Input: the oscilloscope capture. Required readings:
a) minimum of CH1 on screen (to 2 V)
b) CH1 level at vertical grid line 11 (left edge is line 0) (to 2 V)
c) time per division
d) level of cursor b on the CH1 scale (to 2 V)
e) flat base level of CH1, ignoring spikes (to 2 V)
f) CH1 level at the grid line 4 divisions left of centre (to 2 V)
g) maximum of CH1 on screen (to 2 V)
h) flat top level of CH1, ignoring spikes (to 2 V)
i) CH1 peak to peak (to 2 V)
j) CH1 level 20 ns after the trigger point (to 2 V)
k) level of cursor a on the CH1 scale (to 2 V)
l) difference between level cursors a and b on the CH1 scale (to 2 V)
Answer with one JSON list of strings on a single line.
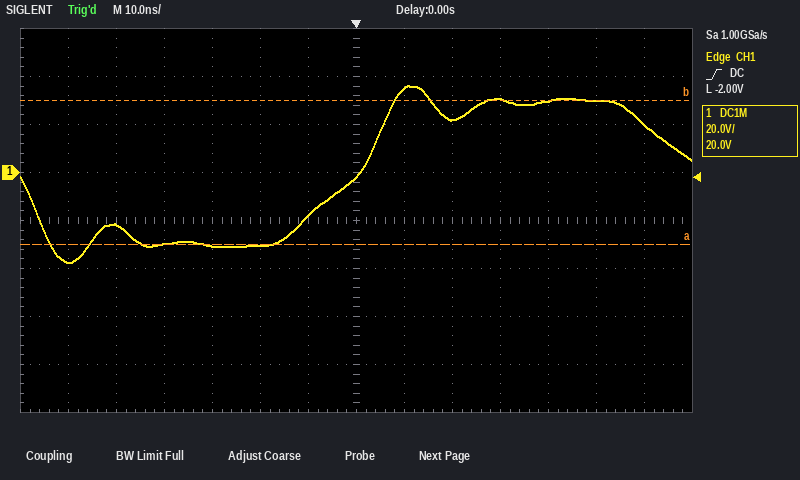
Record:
["-38 V", "30 V", "10 ns", "30 V", "-30 V", "-30 V", "36 V", "30 V", "74 V", "22 V", "-30 V", "60 V"]
